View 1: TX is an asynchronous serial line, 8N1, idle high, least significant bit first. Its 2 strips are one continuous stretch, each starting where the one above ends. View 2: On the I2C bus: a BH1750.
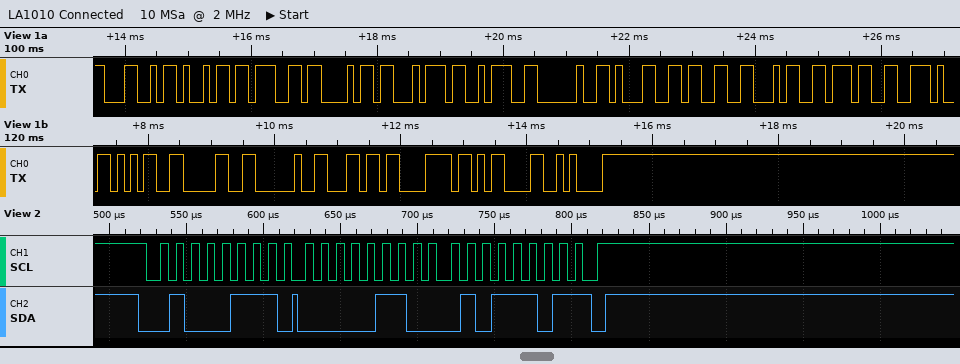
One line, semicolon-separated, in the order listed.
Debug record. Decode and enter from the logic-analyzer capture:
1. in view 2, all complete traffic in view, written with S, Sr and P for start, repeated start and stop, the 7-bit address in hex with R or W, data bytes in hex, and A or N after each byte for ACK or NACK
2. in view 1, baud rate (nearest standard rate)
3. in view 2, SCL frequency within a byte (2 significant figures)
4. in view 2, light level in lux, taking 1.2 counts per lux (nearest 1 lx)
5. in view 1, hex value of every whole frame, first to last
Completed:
S 23R A 06 A 5D N P; 9600 baud; 100 kHz; 1358 lx; 4C 69 67 68 74 3A 20 31 33 34 37 2E 35 30 20 6C 78 0D 0A
